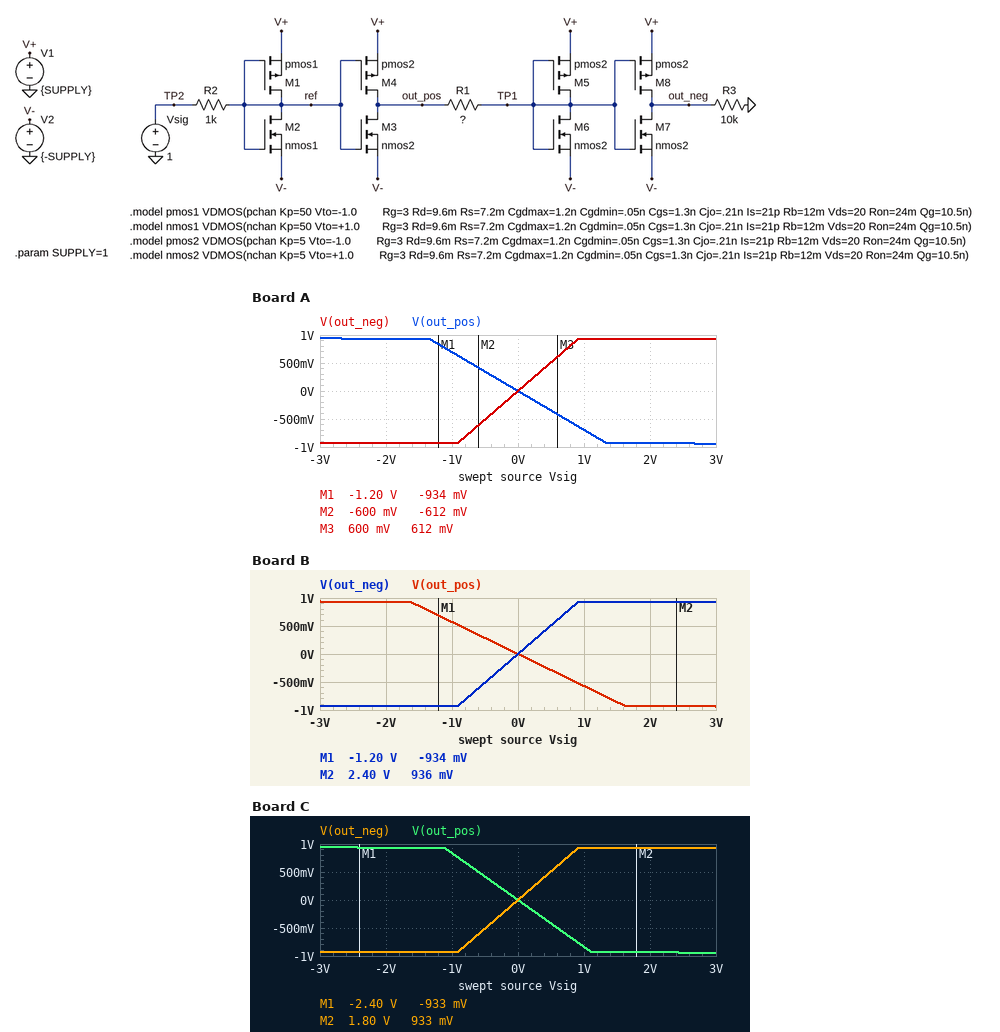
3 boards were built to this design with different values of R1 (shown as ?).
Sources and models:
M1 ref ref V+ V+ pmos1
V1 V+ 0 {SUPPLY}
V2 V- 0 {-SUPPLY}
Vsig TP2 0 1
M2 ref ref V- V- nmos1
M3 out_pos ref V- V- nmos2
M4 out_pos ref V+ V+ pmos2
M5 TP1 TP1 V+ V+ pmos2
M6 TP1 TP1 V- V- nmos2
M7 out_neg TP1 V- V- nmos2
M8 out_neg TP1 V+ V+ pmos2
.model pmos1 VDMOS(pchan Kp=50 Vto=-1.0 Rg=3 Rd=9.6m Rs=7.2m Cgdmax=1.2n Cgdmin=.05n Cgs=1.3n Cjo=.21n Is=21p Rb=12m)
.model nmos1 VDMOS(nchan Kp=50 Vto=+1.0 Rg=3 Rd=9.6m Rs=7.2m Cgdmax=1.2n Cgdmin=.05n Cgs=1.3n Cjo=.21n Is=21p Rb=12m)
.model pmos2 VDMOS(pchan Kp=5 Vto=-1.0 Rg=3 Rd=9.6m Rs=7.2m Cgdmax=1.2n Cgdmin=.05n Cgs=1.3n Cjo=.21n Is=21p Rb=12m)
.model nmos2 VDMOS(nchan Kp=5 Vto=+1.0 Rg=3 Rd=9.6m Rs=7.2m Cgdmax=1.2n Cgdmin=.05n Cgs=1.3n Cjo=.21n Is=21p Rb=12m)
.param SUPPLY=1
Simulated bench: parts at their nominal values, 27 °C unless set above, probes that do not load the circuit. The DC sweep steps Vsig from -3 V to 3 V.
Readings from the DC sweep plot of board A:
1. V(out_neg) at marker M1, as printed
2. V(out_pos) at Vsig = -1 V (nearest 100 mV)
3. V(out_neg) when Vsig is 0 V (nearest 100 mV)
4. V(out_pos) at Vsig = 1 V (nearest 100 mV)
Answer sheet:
-934 mV
700 mV
0 V
-700 mV
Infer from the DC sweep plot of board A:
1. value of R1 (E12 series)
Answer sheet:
6.8 kΩ
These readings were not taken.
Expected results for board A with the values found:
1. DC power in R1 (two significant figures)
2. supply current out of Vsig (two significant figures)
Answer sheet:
71 µW
1.0 mA
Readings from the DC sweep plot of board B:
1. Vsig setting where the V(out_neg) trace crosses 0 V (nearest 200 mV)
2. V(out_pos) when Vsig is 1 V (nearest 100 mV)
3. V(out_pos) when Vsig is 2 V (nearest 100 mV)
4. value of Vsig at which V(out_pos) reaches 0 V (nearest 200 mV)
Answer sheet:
0 V
-600 mV
-900 mV
0 V
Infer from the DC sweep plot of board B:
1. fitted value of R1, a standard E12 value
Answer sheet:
5.6 kΩ
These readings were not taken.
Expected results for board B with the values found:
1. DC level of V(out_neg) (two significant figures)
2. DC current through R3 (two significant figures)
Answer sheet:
930 mV
93 µA
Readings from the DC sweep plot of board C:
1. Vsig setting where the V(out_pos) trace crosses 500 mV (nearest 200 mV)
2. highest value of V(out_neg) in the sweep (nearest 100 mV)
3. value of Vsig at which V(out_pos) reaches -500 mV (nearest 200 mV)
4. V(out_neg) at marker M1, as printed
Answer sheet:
-600 mV
900 mV
600 mV
-933 mV
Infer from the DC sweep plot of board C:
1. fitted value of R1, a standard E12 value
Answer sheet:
8.2 kΩ
